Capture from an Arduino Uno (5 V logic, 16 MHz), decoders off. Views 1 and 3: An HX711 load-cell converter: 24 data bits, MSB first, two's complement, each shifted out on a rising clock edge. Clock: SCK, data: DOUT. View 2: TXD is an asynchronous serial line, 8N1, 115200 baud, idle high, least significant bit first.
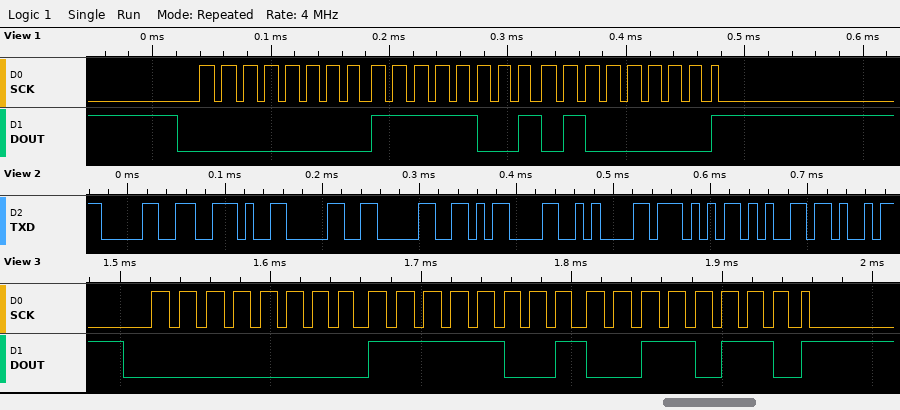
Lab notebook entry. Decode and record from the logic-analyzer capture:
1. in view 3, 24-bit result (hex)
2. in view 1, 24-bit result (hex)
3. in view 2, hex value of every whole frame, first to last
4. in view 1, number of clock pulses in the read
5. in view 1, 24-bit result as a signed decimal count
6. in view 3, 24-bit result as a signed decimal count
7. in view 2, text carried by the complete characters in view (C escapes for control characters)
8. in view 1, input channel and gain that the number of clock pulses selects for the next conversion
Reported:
0x00F936
0x00F940
30 2E 30 30 0D 0A 57 65
25
63808
63798
"0.00\r\nWe"
channel A, gain 128
